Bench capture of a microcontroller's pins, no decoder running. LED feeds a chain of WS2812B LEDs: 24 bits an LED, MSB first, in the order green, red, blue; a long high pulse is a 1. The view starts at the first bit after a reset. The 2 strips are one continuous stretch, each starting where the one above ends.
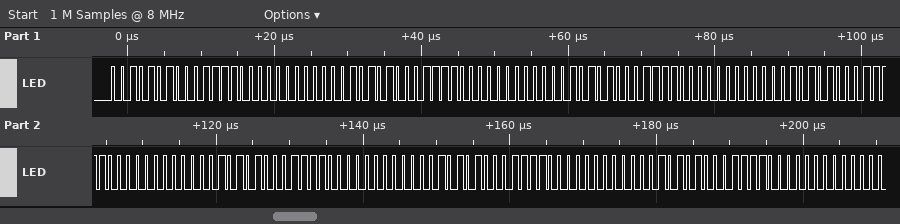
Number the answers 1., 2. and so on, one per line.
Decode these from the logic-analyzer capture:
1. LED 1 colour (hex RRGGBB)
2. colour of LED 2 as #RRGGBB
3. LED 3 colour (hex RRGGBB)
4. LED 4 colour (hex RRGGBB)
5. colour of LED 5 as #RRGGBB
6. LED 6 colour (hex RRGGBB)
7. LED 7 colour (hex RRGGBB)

1. #3C2A00
2. #3C2A00
3. #3C2A00
4. #3C2A00
5. #3C2A00
6. #3C2A00
7. #3C2A00
